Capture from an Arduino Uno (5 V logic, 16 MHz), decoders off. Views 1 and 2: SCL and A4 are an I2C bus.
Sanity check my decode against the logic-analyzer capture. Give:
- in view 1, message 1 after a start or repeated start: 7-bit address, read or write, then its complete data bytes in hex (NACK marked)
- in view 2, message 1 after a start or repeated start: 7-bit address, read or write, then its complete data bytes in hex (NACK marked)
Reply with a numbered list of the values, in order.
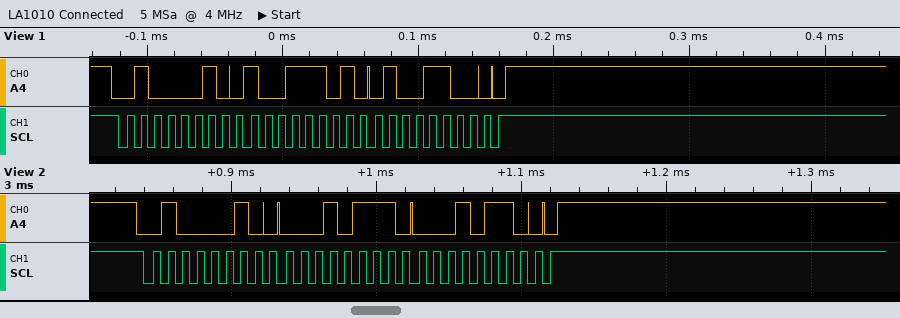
1. 0x21 write: 9D 4C
2. 0x21 write: 17 16
